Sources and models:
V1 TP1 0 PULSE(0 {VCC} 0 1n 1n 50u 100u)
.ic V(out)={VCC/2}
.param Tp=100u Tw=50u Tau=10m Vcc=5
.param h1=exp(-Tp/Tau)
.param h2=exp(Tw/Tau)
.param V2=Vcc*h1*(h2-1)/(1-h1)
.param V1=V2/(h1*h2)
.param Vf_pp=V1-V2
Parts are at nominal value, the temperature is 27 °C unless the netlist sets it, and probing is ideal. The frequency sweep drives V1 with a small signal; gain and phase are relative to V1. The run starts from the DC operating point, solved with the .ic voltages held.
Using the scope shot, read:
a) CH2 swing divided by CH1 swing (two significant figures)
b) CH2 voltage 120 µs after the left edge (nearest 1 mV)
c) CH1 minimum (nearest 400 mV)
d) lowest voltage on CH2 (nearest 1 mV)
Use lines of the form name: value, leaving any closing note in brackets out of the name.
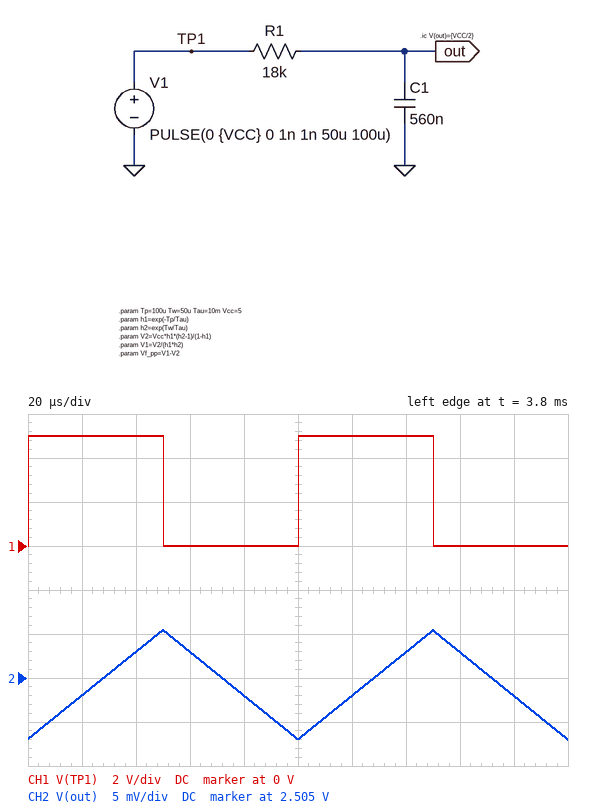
CH2 swing divided by CH1 swing: 0.0025
CH2 voltage 120 µs after the left edge: 2.503 V
CH1 minimum: 0 V
lowest voltage on CH2: 2.498 V
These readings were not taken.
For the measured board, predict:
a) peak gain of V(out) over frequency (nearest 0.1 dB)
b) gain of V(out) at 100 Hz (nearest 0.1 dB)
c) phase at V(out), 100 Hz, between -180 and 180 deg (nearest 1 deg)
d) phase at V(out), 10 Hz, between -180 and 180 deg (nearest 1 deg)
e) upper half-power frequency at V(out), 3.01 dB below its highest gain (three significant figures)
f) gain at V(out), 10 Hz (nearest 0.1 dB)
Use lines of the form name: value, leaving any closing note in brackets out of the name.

peak gain of V(out) over frequency: 0 dB
gain of V(out) at 100 Hz: -16.1 dB
phase at V(out), 100 Hz, between -180 and 180 deg: -81 deg
phase at V(out), 10 Hz, between -180 and 180 deg: -32 deg
upper half-power frequency at V(out), 3.01 dB below its highest gain: 15.8 Hz
gain at V(out), 10 Hz: -1.5 dB
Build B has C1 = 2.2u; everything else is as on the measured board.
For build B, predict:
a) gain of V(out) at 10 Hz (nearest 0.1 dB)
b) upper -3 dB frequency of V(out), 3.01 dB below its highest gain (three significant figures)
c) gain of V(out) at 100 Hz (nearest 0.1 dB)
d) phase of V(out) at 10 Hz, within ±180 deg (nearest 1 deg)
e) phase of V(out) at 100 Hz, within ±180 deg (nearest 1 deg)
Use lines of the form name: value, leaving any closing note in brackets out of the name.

gain of V(out) at 10 Hz: -8.6 dB
upper -3 dB frequency of V(out), 3.01 dB below its highest gain: 4.02 Hz
gain of V(out) at 100 Hz: -27.9 dB
phase of V(out) at 10 Hz, within ±180 deg: -68 deg
phase of V(out) at 100 Hz, within ±180 deg: -88 deg
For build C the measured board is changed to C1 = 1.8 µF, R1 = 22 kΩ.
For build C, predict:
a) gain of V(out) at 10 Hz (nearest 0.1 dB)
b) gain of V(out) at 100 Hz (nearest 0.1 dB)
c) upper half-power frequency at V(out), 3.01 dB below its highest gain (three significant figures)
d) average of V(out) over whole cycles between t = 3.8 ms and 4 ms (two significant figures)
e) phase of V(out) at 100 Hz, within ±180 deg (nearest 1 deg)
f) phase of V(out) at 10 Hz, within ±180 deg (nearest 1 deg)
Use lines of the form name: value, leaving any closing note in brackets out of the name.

gain of V(out) at 10 Hz: -8.6 dB
gain of V(out) at 100 Hz: -27.9 dB
upper half-power frequency at V(out), 3.01 dB below its highest gain: 4.02 Hz
average of V(out) over whole cycles between t = 3.8 ms and 4 ms: 2.5 V
phase of V(out) at 100 Hz, within ±180 deg: -88 deg
phase of V(out) at 10 Hz, within ±180 deg: -68 deg
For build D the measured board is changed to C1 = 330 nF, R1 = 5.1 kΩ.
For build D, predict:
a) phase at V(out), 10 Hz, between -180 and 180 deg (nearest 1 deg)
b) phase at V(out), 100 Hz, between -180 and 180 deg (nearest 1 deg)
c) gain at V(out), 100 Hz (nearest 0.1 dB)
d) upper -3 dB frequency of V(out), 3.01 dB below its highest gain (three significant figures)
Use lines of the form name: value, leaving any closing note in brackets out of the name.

phase at V(out), 10 Hz, between -180 and 180 deg: -6 deg
phase at V(out), 100 Hz, between -180 and 180 deg: -47 deg
gain at V(out), 100 Hz: -3.3 dB
upper -3 dB frequency of V(out), 3.01 dB below its highest gain: 94.6 Hz
